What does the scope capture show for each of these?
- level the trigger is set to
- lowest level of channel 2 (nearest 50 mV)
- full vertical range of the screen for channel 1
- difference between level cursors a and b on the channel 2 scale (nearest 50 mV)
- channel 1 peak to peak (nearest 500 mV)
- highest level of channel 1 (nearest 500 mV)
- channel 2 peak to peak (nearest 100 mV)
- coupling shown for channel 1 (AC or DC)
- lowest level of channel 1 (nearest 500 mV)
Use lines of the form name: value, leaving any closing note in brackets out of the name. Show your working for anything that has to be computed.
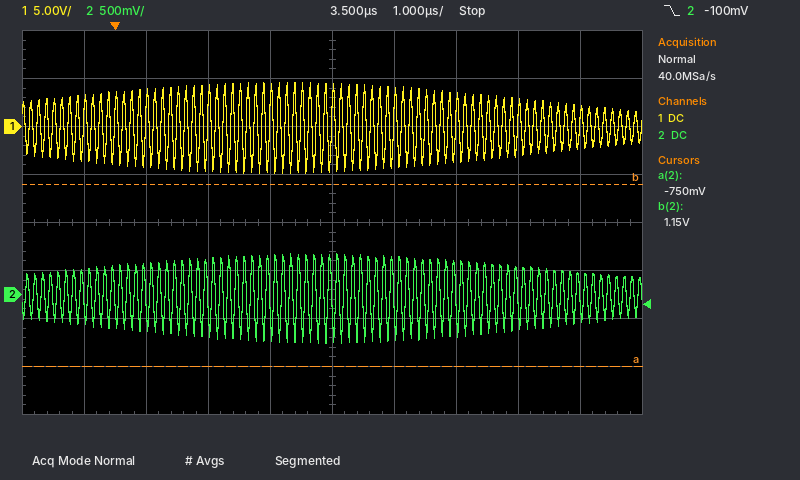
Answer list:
level the trigger is set to: -100 mV
lowest level of channel 2: -500 mV
full vertical range of the screen for channel 1: 40 V
difference between level cursors a and b on the channel 2 scale: 1.90 V
channel 1 peak to peak: 4.5 V − (-5.0 V) = 9.5 V
highest level of channel 1: 4.5 V
channel 2 peak to peak: 900 mV
coupling shown for channel 1: DC
lowest level of channel 1: -5.0 V
